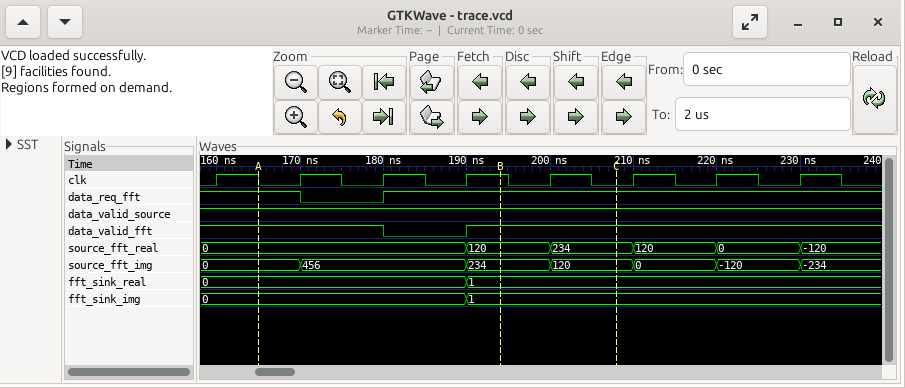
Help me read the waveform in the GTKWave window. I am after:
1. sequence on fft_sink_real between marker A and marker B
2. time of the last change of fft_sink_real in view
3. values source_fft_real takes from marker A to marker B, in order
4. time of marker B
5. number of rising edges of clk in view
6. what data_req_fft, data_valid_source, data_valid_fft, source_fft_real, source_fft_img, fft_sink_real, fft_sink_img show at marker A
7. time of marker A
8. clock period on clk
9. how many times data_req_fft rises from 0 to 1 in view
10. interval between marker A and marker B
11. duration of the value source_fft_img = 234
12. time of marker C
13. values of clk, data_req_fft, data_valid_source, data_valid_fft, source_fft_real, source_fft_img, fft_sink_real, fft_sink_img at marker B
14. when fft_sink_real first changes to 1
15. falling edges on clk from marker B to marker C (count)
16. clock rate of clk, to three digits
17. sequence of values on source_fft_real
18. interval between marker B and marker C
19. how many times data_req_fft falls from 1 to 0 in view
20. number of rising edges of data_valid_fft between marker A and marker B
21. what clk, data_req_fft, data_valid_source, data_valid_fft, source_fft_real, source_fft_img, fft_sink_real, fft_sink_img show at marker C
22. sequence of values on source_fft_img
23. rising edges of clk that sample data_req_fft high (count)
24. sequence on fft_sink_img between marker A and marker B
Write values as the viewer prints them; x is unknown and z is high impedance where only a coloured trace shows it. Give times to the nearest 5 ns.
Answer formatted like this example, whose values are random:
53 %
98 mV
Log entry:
0, 1
190 ns
0, 120
195 ns
8
data_req_fft=1, data_valid_source=1, data_valid_fft=1, source_fft_real=0, source_fft_img=0, fft_sink_real=0, fft_sink_img=0
165 ns
10 ns
1
30 ns
10 ns
210 ns
clk=1, data_req_fft=1, data_valid_source=1, data_valid_fft=1, source_fft_real=120, source_fft_img=234, fft_sink_real=1, fft_sink_img=1
190 ns
2
100 MHz
0, 120, 234, 120, 0, -120
15 ns
1
1
clk=0, data_req_fft=1, data_valid_source=1, data_valid_fft=1, source_fft_real=234, source_fft_img=120, fft_sink_real=1, fft_sink_img=1
0, 456, 234, 120, 0, -120, -234
7
0, 1
